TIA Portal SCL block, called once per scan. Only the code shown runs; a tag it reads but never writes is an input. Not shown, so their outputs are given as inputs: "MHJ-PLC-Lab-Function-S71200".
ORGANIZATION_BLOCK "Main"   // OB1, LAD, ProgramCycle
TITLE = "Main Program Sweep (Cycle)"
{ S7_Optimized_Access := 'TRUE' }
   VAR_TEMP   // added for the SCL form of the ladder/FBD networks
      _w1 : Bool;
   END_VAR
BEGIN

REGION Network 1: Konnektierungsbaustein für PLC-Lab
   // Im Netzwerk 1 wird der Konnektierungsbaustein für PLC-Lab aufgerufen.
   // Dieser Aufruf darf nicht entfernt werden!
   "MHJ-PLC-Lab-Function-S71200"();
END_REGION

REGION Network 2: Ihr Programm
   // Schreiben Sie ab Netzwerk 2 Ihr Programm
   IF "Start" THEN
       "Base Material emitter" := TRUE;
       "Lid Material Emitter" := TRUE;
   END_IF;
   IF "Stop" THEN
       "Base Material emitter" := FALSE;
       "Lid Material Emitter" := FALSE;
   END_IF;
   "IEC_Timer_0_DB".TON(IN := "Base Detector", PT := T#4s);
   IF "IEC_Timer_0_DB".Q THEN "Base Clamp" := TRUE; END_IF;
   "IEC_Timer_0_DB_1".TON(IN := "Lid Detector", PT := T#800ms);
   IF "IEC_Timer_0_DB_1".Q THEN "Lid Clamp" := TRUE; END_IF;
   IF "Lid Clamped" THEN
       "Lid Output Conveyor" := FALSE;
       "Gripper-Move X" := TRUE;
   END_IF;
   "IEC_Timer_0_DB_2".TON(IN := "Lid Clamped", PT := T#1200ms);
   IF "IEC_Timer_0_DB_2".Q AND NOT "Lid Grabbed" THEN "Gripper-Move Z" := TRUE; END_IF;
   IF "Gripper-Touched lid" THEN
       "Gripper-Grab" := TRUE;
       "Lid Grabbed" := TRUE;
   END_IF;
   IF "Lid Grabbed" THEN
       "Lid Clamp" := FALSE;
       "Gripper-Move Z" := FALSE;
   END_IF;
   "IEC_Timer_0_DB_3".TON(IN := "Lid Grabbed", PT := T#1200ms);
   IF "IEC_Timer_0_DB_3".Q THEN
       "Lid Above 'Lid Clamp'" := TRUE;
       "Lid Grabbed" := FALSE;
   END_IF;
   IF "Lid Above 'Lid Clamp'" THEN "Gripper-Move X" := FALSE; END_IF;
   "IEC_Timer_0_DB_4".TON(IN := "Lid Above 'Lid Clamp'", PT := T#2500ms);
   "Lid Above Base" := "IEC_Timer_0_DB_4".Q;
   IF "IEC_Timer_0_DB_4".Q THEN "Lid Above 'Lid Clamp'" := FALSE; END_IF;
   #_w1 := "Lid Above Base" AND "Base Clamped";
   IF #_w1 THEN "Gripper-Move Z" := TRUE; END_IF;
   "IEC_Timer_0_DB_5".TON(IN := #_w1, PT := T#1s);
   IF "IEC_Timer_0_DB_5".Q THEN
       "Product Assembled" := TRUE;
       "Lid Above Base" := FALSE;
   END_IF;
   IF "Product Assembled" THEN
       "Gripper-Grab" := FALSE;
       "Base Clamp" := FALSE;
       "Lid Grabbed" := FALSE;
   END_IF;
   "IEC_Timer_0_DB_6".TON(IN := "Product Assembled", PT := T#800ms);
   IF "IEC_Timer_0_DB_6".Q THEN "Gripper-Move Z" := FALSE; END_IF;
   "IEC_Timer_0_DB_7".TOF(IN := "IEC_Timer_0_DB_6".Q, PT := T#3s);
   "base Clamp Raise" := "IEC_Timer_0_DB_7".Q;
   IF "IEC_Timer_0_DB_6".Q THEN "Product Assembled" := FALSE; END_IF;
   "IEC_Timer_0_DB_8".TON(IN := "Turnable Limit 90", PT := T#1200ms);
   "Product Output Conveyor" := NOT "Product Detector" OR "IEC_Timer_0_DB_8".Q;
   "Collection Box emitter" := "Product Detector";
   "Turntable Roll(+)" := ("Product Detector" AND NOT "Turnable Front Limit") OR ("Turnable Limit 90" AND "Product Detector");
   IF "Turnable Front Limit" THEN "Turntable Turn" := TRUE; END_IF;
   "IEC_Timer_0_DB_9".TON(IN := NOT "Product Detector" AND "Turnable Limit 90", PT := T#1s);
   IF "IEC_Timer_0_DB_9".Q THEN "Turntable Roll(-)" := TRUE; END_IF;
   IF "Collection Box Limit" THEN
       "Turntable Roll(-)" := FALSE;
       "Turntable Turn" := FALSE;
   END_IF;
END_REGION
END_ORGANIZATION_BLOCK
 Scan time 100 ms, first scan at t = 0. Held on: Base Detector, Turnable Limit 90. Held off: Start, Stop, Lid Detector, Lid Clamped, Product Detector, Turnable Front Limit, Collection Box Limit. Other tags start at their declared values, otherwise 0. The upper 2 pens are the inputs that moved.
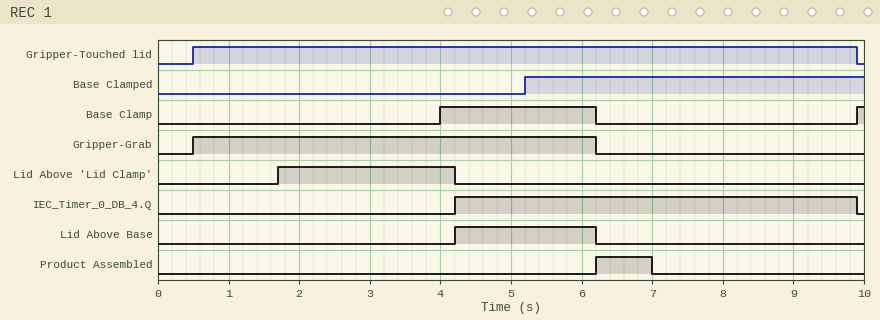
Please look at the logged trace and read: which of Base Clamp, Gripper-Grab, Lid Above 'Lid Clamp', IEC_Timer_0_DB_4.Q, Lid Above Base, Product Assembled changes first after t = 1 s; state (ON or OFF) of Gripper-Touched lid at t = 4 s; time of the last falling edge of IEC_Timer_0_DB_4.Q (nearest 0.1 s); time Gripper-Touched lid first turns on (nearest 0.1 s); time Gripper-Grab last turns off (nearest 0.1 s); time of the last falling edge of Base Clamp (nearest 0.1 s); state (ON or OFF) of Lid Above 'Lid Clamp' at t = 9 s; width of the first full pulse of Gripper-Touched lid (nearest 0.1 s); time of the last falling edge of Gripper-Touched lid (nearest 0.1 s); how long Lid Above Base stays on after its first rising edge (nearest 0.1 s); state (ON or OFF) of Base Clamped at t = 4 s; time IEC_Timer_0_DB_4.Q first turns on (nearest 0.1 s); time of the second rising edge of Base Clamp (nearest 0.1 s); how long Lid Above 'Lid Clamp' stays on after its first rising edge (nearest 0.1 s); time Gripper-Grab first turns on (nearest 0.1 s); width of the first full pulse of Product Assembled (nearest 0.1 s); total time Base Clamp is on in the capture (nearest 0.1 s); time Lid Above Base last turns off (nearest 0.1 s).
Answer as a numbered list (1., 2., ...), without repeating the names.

1. Lid Above 'Lid Clamp'
2. ON
3. 9.9 s
4. 0.5 s
5. 6.2 s
6. 6.2 s
7. OFF
8. 9.4 s
9. 9.9 s
10. 2.0 s
11. OFF
12. 4.2 s
13. 9.9 s
14. 2.5 s
15. 0.5 s
16. 0.8 s
17. 2.3 s
18. 6.2 s
